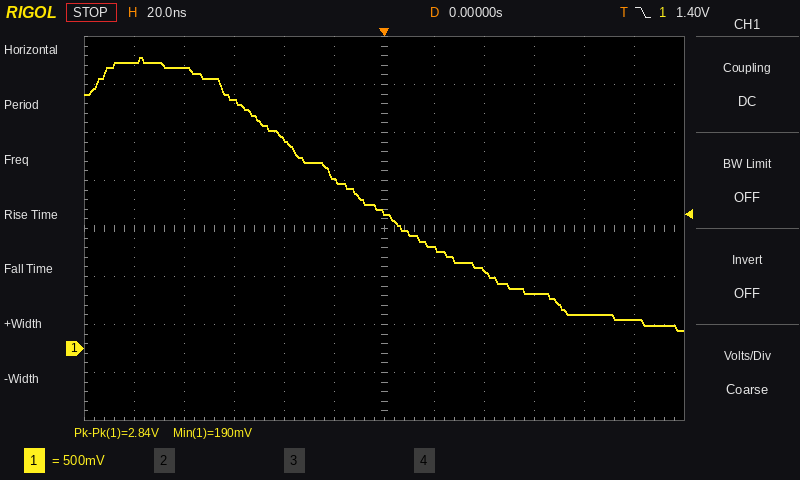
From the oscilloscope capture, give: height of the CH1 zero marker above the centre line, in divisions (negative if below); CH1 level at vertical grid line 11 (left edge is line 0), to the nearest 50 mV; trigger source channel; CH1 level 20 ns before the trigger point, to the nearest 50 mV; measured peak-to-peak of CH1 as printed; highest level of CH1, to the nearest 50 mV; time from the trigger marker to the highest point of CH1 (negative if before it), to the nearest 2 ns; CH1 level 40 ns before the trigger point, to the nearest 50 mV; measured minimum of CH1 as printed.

-2.5 div
300 mV
CH1
1.75 V
2.84 V
3.05 V
-98 ns
2.20 V
190 mV
